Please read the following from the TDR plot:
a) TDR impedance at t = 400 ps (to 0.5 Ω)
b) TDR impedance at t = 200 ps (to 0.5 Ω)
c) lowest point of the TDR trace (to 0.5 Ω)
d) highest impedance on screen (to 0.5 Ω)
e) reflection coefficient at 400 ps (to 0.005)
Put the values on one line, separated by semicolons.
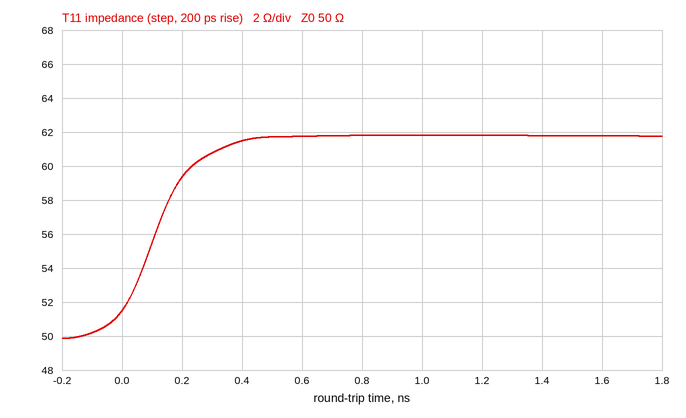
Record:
61.5 Ω; 59.5 Ω; 50.0 Ω; 62.0 Ω; +0.105
